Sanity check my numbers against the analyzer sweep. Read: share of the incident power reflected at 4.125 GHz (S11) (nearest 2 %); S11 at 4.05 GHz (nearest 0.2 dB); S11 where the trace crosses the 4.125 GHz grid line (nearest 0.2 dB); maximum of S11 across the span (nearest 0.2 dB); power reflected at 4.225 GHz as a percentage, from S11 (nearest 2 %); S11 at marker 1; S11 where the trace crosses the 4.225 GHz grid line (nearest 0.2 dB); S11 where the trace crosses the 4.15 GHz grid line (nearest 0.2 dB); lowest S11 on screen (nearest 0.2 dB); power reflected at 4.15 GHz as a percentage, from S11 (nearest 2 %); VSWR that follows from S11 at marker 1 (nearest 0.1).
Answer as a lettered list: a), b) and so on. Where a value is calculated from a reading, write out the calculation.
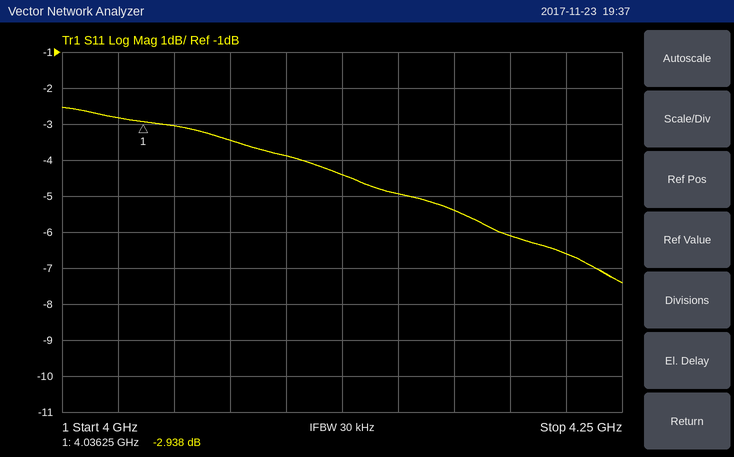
a) 10^(-4.4/10) ≈ 36 %
b) -3.0 dB
c) -4.4 dB
d) -2.6 dB
e) 10^(-6.6/10) ≈ 22 %
f) -2.938 dB
g) -6.6 dB
h) -5.0 dB
i) -7.4 dB
j) 10^(-5/10) ≈ 32 %
k) (1 + 0.7130)/(1 − 0.7130) ≈ 6.0
